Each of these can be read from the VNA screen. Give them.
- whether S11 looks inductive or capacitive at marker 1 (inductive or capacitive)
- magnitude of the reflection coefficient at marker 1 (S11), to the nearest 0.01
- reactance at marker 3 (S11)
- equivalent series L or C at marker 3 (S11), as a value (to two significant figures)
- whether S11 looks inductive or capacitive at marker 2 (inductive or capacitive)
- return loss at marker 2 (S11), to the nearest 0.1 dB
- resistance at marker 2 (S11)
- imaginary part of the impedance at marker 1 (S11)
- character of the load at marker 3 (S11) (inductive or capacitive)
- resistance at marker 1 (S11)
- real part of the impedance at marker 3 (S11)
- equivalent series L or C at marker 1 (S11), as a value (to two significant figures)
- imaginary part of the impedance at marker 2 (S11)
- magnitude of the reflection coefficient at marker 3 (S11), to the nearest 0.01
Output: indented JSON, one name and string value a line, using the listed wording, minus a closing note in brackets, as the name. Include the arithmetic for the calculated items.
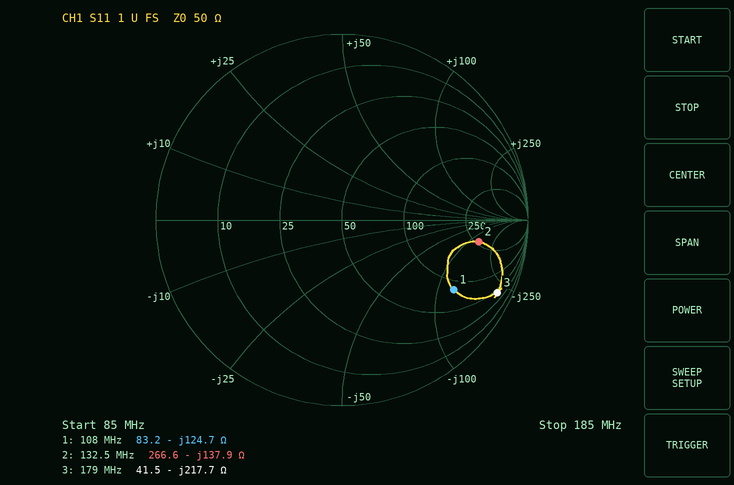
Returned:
{
  "whether S11 looks inductive or capacitive at marker 1": "capacitive",
  "magnitude of the reflection coefficient at marker 1 (S11), to the nearest 0.01": "0.71",
  "reactance at marker 3": "-217.7 Ω",
  "equivalent series L or C at marker 3 (S11), as a value": "C = 1/(2π × 179 MHz × 217.7 Ω) ≈ 4.1 pF",
  "whether S11 looks inductive or capacitive at marker 2": "capacitive",
  "return loss at marker 2 (S11), to the nearest 0.1 dB": "2.6 dB",
  "resistance at marker 2": "266.6 Ω",
  "imaginary part of the impedance at marker 1": "-124.7 Ω",
  "character of the load at marker 3 (S11)": "capacitive",
  "resistance at marker 1": "83.2 Ω",
  "real part of the impedance at marker 3": "41.5 Ω",
  "equivalent series L or C at marker 1 (S11), as a value": "C = 1/(2π × 108 MHz × 124.7 Ω) ≈ 12 pF",
  "imaginary part of the impedance at marker 2": "-137.9 Ω",
  "magnitude of the reflection coefficient at marker 3 (S11), to the nearest 0.01": "0.92"
}
